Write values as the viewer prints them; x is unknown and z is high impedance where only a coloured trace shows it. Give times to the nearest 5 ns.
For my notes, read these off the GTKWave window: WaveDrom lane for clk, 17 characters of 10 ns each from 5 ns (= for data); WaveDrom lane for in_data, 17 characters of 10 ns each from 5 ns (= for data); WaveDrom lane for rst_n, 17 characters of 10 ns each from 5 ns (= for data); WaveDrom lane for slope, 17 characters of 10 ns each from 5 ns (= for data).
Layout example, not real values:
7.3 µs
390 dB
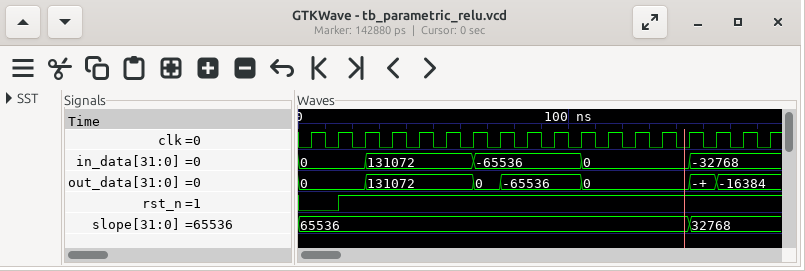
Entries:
{name: 'clk', wave: 'p................'}
{name: 'in_data', wave: '=.=...=...=...=..', data: '0 131072 -65536 0 -32768'}
{name: 'rst_n', wave: '01...............'}
{name: 'slope', wave: '=.............=..', data: '65536 32768'}
